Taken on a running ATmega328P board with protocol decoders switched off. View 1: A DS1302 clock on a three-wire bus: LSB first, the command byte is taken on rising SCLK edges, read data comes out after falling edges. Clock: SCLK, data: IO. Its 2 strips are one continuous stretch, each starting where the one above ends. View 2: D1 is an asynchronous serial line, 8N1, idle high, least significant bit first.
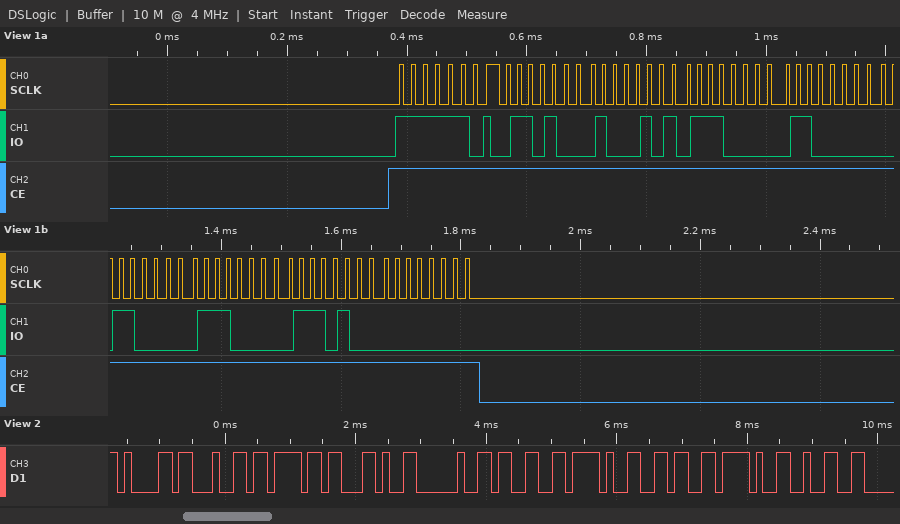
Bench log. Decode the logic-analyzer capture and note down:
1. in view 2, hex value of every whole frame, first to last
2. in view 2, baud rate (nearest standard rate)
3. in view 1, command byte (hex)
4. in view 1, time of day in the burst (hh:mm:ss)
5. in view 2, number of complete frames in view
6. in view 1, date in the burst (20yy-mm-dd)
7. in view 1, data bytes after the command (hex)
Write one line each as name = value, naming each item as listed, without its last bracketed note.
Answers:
in view 2, hex value of every whole frame, first to last = 61 64 6F 2C 20 33 2F 36 2F 32
in view 2, baud rate = 9600 baud
in view 1, command byte = 0xBF
in view 1, time of day in the burst = 07:51:16
in view 2, number of complete frames in view = 10
in view 1, date in the burst = 2017-06-03
in view 1, data bytes after the command = 16 51 07 03 06 07 17 00
